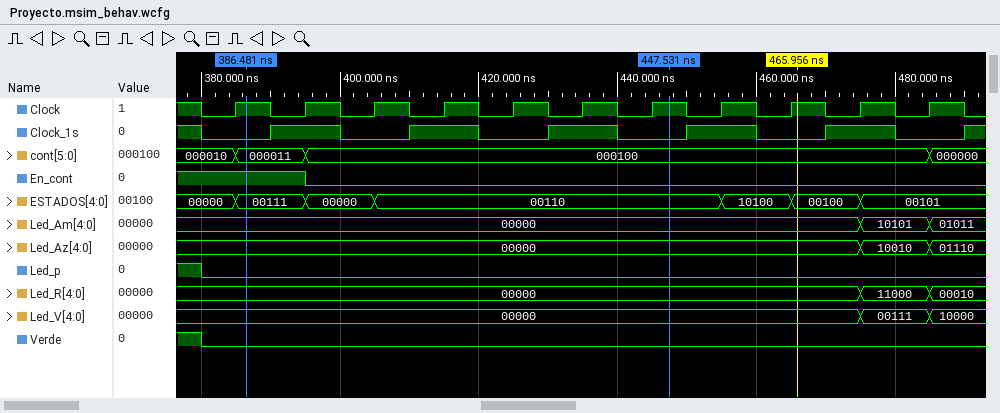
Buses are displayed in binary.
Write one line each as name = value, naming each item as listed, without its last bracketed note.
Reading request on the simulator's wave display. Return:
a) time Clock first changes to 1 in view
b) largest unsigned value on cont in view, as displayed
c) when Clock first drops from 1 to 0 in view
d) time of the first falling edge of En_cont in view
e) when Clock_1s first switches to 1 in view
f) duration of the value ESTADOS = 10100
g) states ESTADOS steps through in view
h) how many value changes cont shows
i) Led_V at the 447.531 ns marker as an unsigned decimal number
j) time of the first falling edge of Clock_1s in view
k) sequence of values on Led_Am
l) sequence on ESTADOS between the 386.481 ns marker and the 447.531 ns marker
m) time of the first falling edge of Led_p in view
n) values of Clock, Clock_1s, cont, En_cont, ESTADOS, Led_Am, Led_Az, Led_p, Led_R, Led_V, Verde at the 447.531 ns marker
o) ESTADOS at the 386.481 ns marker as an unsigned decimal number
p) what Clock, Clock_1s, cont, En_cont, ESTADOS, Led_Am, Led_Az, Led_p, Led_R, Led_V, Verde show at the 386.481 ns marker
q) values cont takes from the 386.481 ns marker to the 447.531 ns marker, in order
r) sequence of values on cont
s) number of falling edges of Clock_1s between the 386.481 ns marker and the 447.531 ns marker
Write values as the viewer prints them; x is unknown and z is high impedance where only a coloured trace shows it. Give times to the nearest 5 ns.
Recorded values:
time Clock first changes to 1 in view = 385 ns
largest unsigned value on cont in view, as displayed = 000100
when Clock first drops from 1 to 0 in view = 380 ns
time of the first falling edge of En_cont in view = 395 ns
when Clock_1s first switches to 1 in view = 390 ns
duration of the value ESTADOS = 10100 = 10 ns
states ESTADOS steps through in view = 00000, 00111, 00000, 00110, 10100, 00100, 00101
how many value changes cont shows = 3
Led_V at the 447.531 ns marker as an unsigned decimal number = 0
time of the first falling edge of Clock_1s in view = 380 ns
sequence of values on Led_Am = 00000, 10101, 01011
sequence on ESTADOS between the 386.481 ns marker and the 447.531 ns marker = 00111, 00000, 00110
time of the first falling edge of Led_p in view = 380 ns
values of Clock, Clock_1s, cont, En_cont, ESTADOS, Led_Am, Led_Az, Led_p, Led_R, Led_V, Verde at the 447.531 ns marker = Clock=1, Clock_1s=0, cont=000100, En_cont=0, ESTADOS=00110, Led_Am=00000, Led_Az=00000, Led_p=0, Led_R=00000, Led_V=00000, Verde=0
ESTADOS at the 386.481 ns marker as an unsigned decimal number = 7
what Clock, Clock_1s, cont, En_cont, ESTADOS, Led_Am, Led_Az, Led_p, Led_R, Led_V, Verde show at the 386.481 ns marker = Clock=1, Clock_1s=0, cont=000011, En_cont=1, ESTADOS=00111, Led_Am=00000, Led_Az=00000, Led_p=0, Led_R=00000, Led_V=00000, Verde=0
values cont takes from the 386.481 ns marker to the 447.531 ns marker, in order = 000011, 000100
sequence of values on cont = 000010, 000011, 000100, 000000
number of falling edges of Clock_1s between the 386.481 ns marker and the 447.531 ns marker = 3
